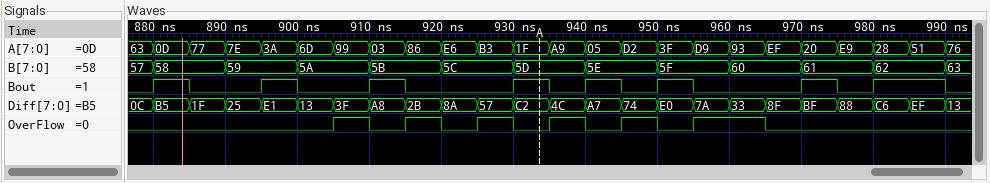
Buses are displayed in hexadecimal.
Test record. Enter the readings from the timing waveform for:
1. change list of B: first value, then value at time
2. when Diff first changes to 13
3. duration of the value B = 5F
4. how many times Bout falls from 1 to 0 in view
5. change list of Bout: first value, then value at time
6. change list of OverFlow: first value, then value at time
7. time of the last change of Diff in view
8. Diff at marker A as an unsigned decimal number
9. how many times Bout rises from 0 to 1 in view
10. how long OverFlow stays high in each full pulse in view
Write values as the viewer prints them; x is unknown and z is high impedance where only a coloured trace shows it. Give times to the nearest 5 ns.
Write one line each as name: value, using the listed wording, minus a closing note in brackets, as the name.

change list of B: first value, then value at time: 57, 58 at 880 ns, 59 at 890 ns, 5A at 900 ns, 5B at 910 ns, 5C at 920 ns, 5D at 930 ns, 5E at 940 ns, 5F at 950 ns, 60 at 960 ns, 61 at 970 ns, 62 at 980 ns, 63 at 990 ns
when Diff first changes to 13: 900 ns
duration of the value B = 5F: 10 ns
how many times Bout falls from 1 to 0 in view: 8
change list of Bout: first value, then value at time: 0, 1 at 880 ns, 0 at 885 ns, 1 at 895 ns, 0 at 900 ns, 1 at 910 ns, 0 at 915 ns, 1 at 930 ns, 0 at 935 ns, 1 at 940 ns, 0 at 945 ns, 1 at 950 ns, 0 at 955 ns, 1 at 970 ns, 0 at 975 ns, 1 at 980 ns, 0 at 990 ns
change list of OverFlow: first value, then value at time: 0, 1 at 905 ns, 0 at 910 ns, 1 at 915 ns, 0 at 920 ns, 1 at 925 ns, 0 at 930 ns, 1 at 935 ns, 0 at 940 ns, 1 at 945 ns, 0 at 950 ns, 1 at 955 ns, 0 at 965 ns
time of the last change of Diff in view: 990 ns
Diff at marker A as an unsigned decimal number: 194
how many times Bout rises from 0 to 1 in view: 8
how long OverFlow stays high in each full pulse in view: 5 ns, 5 ns, 5 ns, 5 ns, 5 ns, 10 ns
